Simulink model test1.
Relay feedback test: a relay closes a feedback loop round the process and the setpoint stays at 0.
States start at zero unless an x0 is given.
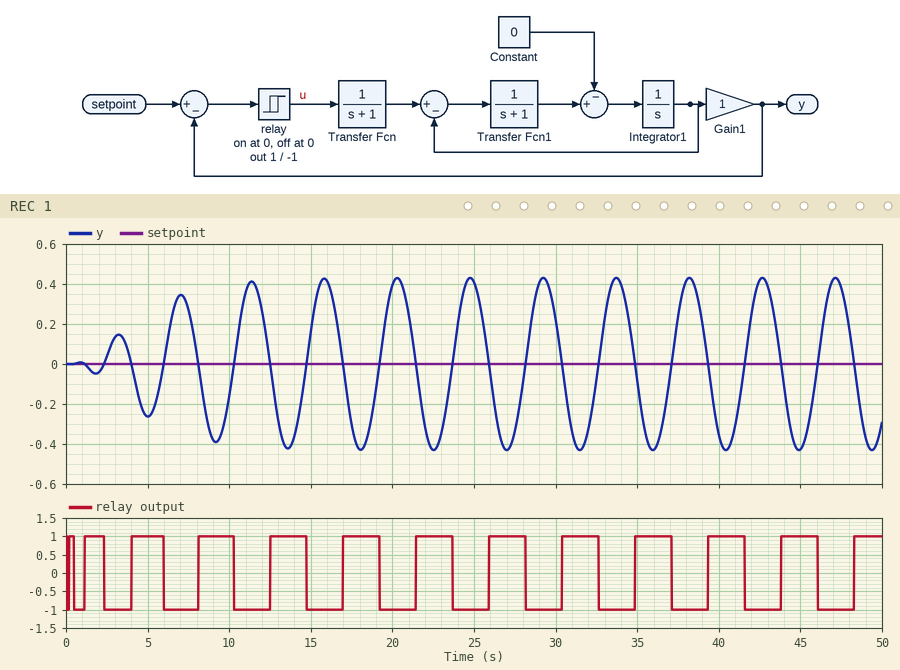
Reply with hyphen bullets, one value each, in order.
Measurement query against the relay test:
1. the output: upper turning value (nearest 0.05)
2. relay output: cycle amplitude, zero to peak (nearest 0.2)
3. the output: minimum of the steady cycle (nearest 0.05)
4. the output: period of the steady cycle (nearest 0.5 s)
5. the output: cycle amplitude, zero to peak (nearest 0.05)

- 0.45
- 1.0
- -0.45
- 4.5 s
- 0.45
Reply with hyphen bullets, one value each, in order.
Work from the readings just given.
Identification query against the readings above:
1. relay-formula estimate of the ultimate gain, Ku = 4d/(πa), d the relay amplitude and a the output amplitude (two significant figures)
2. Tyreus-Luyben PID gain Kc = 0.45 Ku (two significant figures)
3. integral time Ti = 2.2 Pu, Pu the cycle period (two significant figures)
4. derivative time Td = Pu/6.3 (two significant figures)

- 2.8
- 1.3
- 9.9 s
- 0.71 s
